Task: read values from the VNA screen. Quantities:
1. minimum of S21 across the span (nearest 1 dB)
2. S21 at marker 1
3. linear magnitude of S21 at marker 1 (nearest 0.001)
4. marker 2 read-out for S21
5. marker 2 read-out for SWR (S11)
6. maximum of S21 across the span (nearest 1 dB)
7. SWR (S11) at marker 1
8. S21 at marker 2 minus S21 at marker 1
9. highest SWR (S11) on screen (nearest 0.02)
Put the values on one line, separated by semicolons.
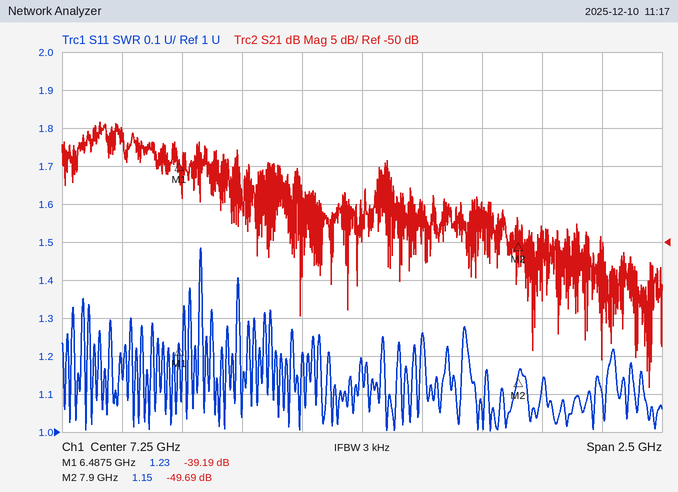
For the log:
-69 dB; -39.19 dB; 0.011; -49.69 dB; 1.15; -34 dB; 1.23; -10.50 dB; 1.48
